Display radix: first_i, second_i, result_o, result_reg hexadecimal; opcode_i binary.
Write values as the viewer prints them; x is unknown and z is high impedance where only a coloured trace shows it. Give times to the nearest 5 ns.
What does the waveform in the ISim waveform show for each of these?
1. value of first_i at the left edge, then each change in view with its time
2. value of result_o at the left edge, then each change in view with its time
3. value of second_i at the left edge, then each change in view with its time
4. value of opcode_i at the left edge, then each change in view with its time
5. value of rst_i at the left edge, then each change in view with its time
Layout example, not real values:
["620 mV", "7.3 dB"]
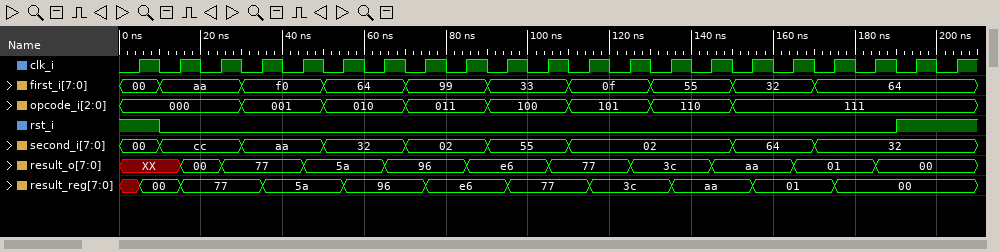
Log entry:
["00, aa at 10 ns, f0 at 30 ns, 64 at 50 ns, 99 at 70 ns, 33 at 90 ns, 0f at 110 ns, 55 at 130 ns, 32 at 150 ns, 64 at 170 ns", "XX, 00 at 15 ns, 77 at 25 ns, 5a at 45 ns, 96 at 65 ns, e6 at 85 ns, 77 at 105 ns, 3c at 125 ns, aa at 145 ns, 01 at 165 ns, 00 at 185 ns", "00, cc at 10 ns, aa at 30 ns, 32 at 50 ns, 02 at 70 ns, 55 at 90 ns, 02 at 110 ns, 64 at 150 ns, 32 at 170 ns", "000, 001 at 30 ns, 010 at 50 ns, 011 at 70 ns, 100 at 90 ns, 101 at 110 ns, 110 at 130 ns, 111 at 150 ns", "1, 0 at 10 ns, 1 at 190 ns"]
